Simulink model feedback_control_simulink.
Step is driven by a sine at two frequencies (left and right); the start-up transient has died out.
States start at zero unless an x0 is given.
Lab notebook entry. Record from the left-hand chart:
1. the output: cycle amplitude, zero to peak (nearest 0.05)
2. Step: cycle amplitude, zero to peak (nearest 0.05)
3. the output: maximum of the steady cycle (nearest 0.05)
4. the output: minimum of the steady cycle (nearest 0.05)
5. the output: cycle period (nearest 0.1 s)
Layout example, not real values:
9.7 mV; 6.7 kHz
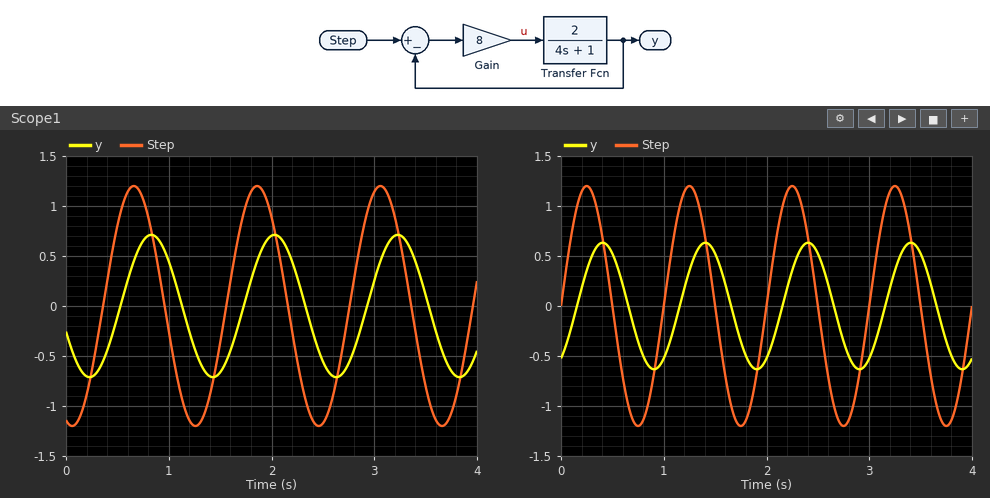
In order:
0.70; 1.20; 0.70; -0.70; 1.2 s
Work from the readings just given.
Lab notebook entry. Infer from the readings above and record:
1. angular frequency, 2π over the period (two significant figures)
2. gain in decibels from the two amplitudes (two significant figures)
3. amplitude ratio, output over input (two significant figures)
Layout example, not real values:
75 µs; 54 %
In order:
5.2 rad/s; -4.7 dB; 0.58
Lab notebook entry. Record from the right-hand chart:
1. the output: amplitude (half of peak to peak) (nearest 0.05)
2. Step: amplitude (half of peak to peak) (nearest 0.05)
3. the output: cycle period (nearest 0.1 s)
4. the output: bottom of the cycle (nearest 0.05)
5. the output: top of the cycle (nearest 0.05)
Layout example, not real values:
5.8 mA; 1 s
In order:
0.65; 1.20; 1.0 s; -0.65; 0.65
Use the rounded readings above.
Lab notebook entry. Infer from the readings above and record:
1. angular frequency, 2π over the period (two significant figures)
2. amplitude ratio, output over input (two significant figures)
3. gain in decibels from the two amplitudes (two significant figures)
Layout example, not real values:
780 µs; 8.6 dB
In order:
6.3 rad/s; 0.54; -5.3 dB
